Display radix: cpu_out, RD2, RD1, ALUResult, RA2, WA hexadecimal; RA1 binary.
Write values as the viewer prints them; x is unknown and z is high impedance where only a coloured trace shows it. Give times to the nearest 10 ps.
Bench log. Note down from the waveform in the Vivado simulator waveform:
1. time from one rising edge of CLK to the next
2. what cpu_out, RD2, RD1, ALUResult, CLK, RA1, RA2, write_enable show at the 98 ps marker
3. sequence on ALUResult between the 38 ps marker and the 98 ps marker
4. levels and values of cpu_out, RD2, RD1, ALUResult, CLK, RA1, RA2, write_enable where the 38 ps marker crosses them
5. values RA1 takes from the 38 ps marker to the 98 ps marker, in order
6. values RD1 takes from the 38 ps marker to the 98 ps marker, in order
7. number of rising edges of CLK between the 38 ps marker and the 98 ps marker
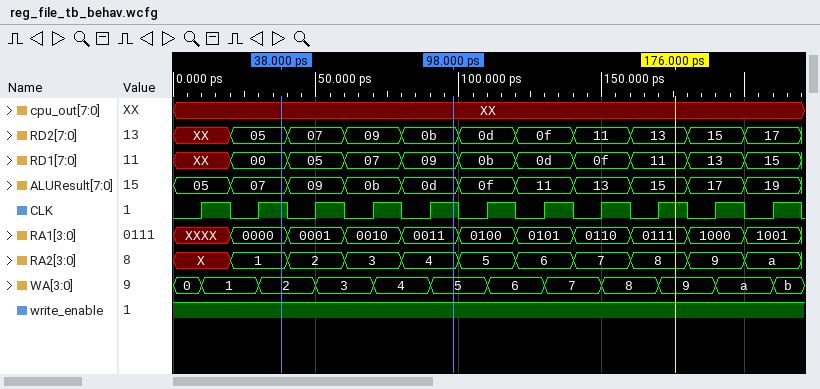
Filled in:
20 ps
cpu_out=XX, RD2=0b, RD1=09, ALUResult=0d, CLK=1, RA1=0011, RA2=4, write_enable=1
07, 09, 0b, 0d
cpu_out=XX, RD2=05, RD1=00, ALUResult=07, CLK=1, RA1=0000, RA2=1, write_enable=1
0000, 0001, 0010, 0011
00, 05, 07, 09
3
